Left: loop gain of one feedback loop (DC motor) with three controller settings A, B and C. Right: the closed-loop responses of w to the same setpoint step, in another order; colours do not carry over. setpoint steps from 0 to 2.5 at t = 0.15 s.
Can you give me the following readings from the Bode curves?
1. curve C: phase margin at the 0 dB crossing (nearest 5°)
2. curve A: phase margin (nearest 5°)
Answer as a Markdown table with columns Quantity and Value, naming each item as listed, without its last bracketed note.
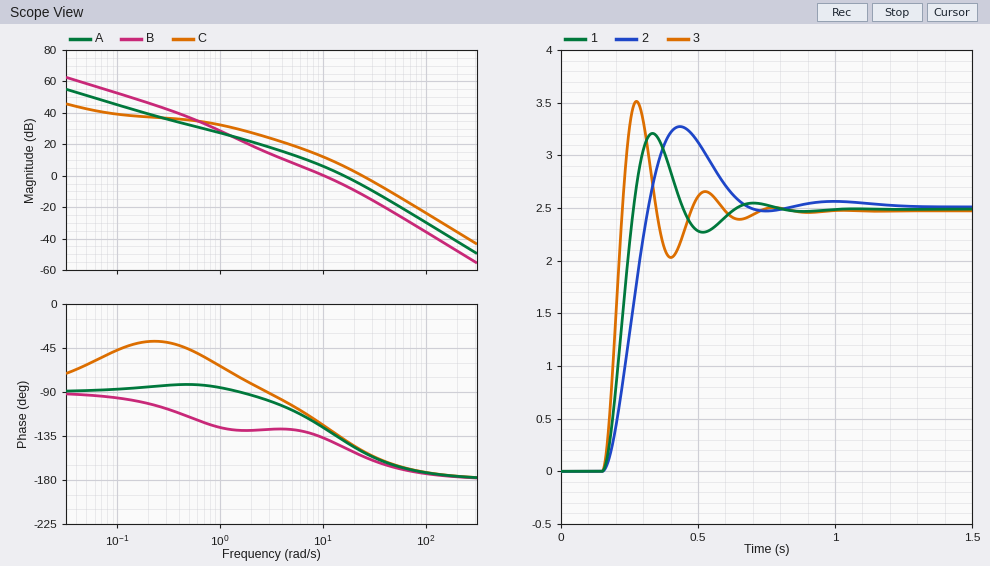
| Quantity | Value |
|---|---|
| curve C: phase margin at the 0 dB crossing | 30° |
| curve A: phase margin | 40° |
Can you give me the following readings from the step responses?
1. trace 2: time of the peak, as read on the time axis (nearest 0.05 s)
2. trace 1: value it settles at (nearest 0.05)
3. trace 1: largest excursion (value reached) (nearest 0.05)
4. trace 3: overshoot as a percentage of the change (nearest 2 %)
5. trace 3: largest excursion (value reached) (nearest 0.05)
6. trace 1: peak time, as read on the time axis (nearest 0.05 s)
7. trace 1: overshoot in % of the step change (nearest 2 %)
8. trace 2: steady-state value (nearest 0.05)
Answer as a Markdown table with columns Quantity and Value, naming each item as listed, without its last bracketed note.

| Quantity | Value |
|---|---|
| trace 2: time of the peak, as read on the time axis | 0.45 s |
| trace 1: value it settles at | 2.50 |
| trace 1: largest excursion (value reached) | 3.20 |
| trace 3: overshoot as a percentage of the change | 42 % |
| trace 3: largest excursion (value reached) | 3.50 |
| trace 1: peak time, as read on the time axis | 0.35 s |
| trace 1: overshoot in % of the step change | 28 % |
| trace 2: steady-state value | 2.50 |
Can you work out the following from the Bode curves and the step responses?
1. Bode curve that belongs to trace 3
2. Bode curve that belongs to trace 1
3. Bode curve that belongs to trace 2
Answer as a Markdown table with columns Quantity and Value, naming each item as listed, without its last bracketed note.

| Quantity | Value |
|---|---|
| Bode curve that belongs to trace 3 | C |
| Bode curve that belongs to trace 1 | A |
| Bode curve that belongs to trace 2 | B |
